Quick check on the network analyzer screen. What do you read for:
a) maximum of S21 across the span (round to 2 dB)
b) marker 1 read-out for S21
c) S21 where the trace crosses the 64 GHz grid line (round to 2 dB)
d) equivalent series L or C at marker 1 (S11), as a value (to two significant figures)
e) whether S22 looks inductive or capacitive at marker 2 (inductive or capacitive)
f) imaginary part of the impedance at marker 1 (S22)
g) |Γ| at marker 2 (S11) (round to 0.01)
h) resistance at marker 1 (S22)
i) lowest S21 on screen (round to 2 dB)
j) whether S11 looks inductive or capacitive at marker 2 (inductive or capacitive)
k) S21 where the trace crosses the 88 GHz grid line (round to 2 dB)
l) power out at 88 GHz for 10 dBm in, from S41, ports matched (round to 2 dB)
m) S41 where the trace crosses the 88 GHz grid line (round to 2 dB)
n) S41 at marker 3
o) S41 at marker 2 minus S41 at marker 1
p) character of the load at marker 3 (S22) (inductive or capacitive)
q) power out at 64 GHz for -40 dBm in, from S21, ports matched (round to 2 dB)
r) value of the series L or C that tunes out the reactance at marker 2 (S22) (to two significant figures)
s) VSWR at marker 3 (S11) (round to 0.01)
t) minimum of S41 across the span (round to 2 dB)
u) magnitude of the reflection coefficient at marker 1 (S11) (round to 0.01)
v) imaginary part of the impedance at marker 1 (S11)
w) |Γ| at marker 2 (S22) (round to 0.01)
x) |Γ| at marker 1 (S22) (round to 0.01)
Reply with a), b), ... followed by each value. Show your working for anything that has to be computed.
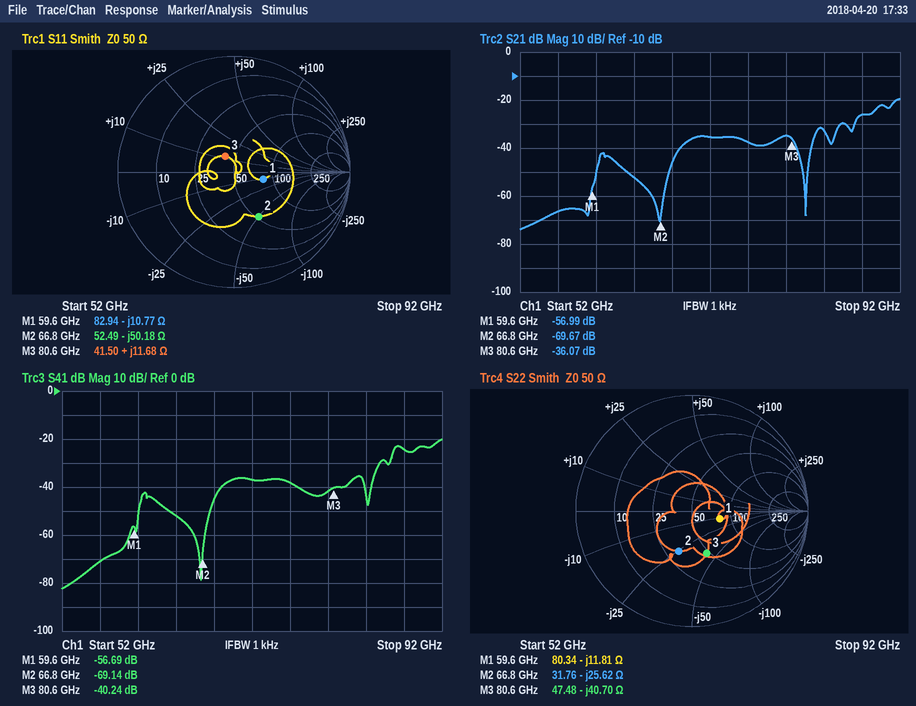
a) -20 dB
b) -56.99 dB
c) -52 dB
d) C = 1/(2π × 59.6 GHz × 10.77 Ω) ≈ 248 fF, so 250 fF to two significant figures
e) capacitive
f) -11.81 Ω
g) 0.44
h) 80.34 Ω
i) -74 dB
j) capacitive
k) -26 dB
l) 10 dBm + (-24 dB) = -14 dBm
m) -24 dB
n) -40.24 dB
o) -69.14 − (-56.69) = -12.45 dB
p) capacitive
q) -40 dBm + (-52 dB) = -92 dBm
r) L = 25.62 Ω/(2π × 66.8 GHz) ≈ 61 pH
s) 1.37
t) -82 dB
u) 0.26
v) -10.77 Ω
w) 0.37
x) 0.25
